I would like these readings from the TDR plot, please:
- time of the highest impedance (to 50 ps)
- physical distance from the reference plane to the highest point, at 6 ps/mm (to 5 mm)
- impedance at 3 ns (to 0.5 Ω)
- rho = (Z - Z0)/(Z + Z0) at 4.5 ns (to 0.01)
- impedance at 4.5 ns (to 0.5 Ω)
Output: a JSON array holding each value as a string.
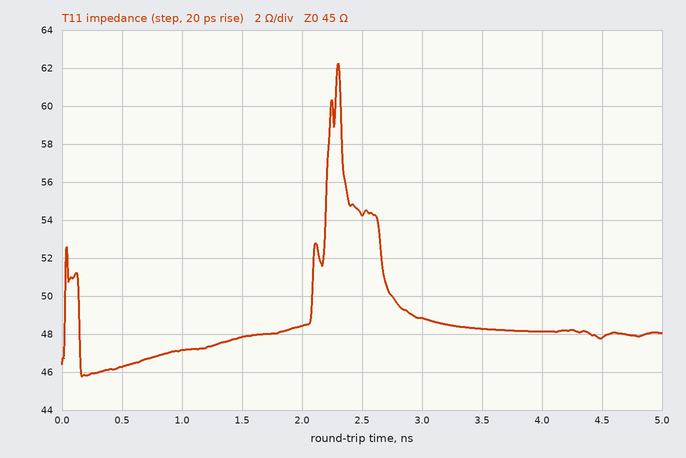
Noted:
["2.30 ns", "190 mm", "49.0 Ω", "+0.03", "48.0 Ω"]
